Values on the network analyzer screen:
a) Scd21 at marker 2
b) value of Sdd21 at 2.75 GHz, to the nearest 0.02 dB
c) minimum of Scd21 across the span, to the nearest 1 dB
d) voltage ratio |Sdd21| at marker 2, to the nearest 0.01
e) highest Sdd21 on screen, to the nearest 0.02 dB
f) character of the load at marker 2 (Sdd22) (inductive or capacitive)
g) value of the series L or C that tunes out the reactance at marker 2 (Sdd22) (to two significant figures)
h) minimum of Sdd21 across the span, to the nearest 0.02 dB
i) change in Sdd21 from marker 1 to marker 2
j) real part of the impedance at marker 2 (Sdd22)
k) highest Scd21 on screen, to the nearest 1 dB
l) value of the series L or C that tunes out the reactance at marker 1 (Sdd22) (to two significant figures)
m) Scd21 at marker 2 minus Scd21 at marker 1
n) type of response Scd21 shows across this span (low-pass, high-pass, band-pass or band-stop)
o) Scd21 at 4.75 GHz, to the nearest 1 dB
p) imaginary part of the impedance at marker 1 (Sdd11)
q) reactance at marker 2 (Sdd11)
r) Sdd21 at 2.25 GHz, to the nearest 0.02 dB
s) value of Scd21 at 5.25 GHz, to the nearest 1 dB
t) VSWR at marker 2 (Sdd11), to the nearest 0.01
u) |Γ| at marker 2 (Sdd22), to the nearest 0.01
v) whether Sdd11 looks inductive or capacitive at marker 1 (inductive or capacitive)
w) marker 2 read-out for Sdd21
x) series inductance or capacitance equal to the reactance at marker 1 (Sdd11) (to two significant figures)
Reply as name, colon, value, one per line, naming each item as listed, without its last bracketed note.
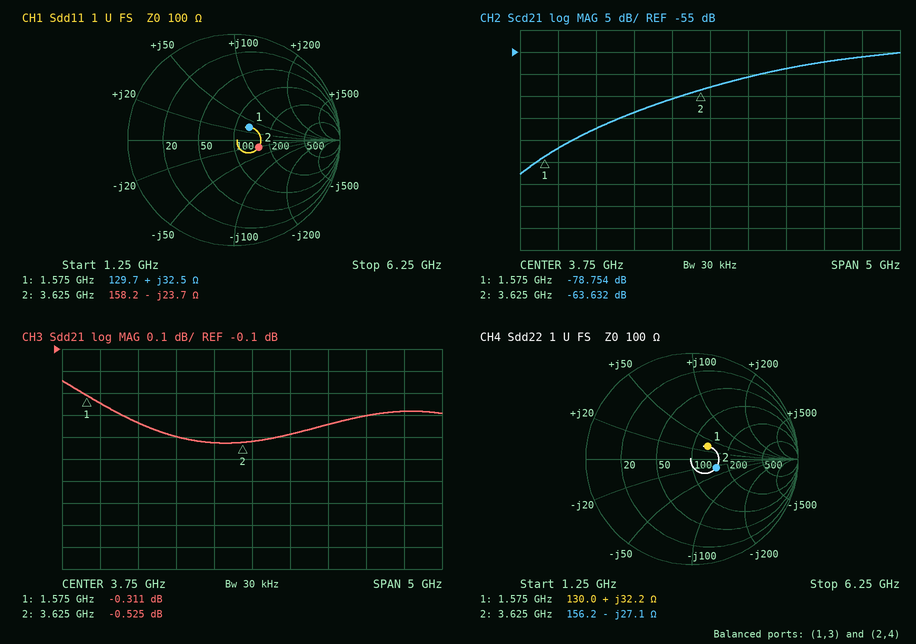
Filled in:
Scd21 at marker 2: -63.632 dB
value of Sdd21 at 2.75 GHz, to the nearest 0.02 dB: -0.50 dB
minimum of Scd21 across the span, to the nearest 1 dB: -83 dB
voltage ratio |Sdd21| at marker 2, to the nearest 0.01: 0.94
highest Sdd21 on screen, to the nearest 0.02 dB: -0.24 dB
character of the load at marker 2 (Sdd22): capacitive
value of the series L or C that tunes out the reactance at marker 2 (Sdd22): 1.2 nH
minimum of Sdd21 across the span, to the nearest 0.02 dB: -0.52 dB
change in Sdd21 from marker 1 to marker 2: -0.214 dB
real part of the impedance at marker 2: 156.2 Ω
highest Scd21 on screen, to the nearest 1 dB: -55 dB
value of the series L or C that tunes out the reactance at marker 1 (Sdd22): 3.1 pF
Scd21 at marker 2 minus Scd21 at marker 1: 15.122 dB
type of response Scd21 shows across this span: high-pass
Scd21 at 4.75 GHz, to the nearest 1 dB: -59 dB
imaginary part of the impedance at marker 1: +32.5 Ω
reactance at marker 2: -23.7 Ω
Sdd21 at 2.25 GHz, to the nearest 0.02 dB: -0.44 dB
value of Scd21 at 5.25 GHz, to the nearest 1 dB: -57 dB
VSWR at marker 2 (Sdd11), to the nearest 0.01: 1.64
|Γ| at marker 2 (Sdd22), to the nearest 0.01: 0.24
whether Sdd11 looks inductive or capacitive at marker 1: inductive
marker 2 read-out for Sdd21: -0.525 dB
series inductance or capacitance equal to the reactance at marker 1 (Sdd11): 3.3 nH
